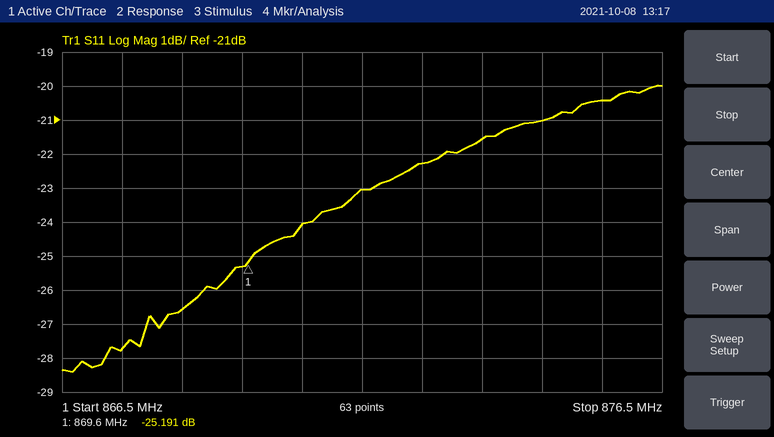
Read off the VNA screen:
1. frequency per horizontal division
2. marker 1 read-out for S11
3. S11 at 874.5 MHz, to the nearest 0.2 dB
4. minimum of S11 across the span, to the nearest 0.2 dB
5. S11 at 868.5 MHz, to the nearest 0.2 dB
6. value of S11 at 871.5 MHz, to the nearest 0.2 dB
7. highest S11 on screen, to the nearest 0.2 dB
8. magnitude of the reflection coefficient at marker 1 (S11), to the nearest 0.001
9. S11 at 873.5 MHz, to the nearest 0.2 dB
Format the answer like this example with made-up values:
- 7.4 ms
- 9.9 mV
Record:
- 1 MHz
- -25.191 dB
- -21.0 dB
- -28.4 dB
- -26.6 dB
- -23.0 dB
- -20.0 dB
- 0.055
- -21.6 dB
